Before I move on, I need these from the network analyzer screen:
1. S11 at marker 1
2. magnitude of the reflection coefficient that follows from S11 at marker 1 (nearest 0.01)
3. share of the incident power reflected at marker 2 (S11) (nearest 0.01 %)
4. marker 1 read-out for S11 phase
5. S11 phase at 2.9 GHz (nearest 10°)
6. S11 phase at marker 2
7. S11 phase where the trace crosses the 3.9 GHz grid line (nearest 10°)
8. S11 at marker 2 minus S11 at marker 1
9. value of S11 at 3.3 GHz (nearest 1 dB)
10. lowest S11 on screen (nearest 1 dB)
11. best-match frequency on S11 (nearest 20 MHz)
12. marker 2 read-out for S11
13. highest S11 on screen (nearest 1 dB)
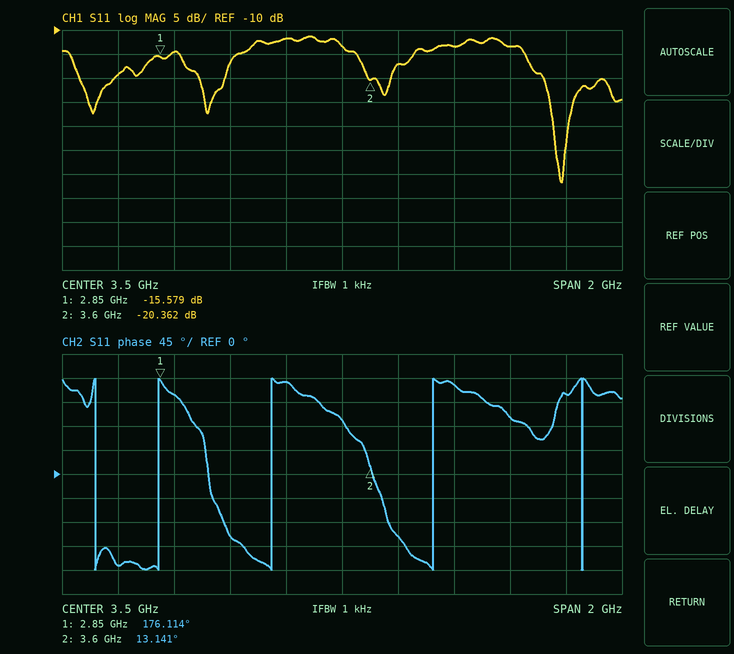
-15.579 dB
0.17
0.92 %
176.114°
150°
13.141°
170°
-4.783 dB
-12 dB
-42 dB
4.28 GHz
-20.362 dB
-11 dB
